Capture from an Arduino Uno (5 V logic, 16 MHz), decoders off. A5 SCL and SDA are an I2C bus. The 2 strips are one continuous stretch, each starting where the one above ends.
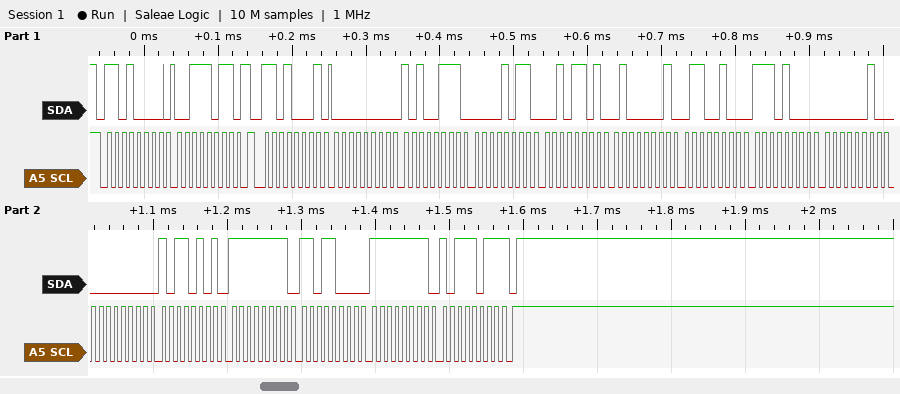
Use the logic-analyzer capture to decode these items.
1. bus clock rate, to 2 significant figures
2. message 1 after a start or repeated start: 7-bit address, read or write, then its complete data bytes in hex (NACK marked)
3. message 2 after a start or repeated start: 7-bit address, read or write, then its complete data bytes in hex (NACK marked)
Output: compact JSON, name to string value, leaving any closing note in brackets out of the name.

{"bus clock rate, to 2 significant figures": "100 kHz", "message 1 after a start or repeated start: 7-bit address, read or write, then its complete data bytes in hex": "0x68 write: 3B", "message 2 after a start or repeated start: 7-bit address, read or write, then its complete data bytes in hex": "0x68 read: 00 A7 0B 2D 41 64 E8 02 00 B5 FF D8 FF BB NACK"}
